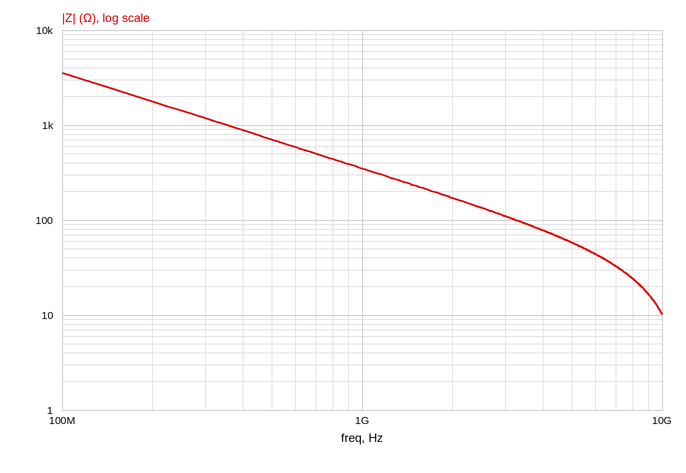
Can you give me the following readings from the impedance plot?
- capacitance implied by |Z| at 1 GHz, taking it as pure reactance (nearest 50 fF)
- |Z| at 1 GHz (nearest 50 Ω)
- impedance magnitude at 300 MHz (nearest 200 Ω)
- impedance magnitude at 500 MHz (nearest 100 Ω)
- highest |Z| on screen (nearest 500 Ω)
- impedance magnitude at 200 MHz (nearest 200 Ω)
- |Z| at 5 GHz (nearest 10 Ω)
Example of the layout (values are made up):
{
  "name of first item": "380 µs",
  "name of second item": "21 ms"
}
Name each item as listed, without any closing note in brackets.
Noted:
{
  "capacitance implied by |Z| at 1 GHz, taking it as pure reactance": "450 fF",
  "|Z| at 1 GHz": "350 Ω",
  "impedance magnitude at 300 MHz": "1.2 kΩ",
  "impedance magnitude at 500 MHz": "700 Ω",
  "highest |Z| on screen": "3.5 kΩ",
  "impedance magnitude at 200 MHz": "1.8 kΩ",
  "|Z| at 5 GHz": "60 Ω"
}
